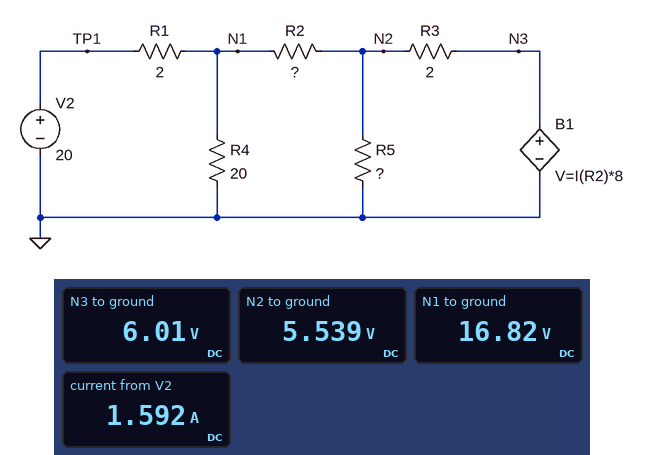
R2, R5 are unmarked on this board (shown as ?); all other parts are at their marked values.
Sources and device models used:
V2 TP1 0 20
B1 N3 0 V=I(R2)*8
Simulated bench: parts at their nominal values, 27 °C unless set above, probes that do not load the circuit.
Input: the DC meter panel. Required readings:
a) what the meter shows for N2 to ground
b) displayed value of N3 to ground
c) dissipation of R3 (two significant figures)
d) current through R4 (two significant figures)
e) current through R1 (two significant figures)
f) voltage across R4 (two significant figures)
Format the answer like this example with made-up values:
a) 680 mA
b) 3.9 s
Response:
a) 5.539 V
b) 6.01 V
c) 110 mW
d) 840 mA
e) 1.6 A
f) 17 V
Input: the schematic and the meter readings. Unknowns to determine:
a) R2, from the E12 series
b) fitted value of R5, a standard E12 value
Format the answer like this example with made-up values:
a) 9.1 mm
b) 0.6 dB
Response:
a) 15 Ω
b) 5.6 Ω
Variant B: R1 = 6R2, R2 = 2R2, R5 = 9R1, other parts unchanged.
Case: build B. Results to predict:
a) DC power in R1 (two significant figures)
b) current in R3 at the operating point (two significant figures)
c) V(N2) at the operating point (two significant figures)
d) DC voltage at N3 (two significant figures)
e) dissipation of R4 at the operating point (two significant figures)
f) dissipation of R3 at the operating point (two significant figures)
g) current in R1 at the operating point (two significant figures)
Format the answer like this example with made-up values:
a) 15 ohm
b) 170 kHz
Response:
a) 15 W
b) 100 mA
c) 8.3 V
d) 8.1 V
e) 5.5 W
f) 20 mW
g) 1.5 A
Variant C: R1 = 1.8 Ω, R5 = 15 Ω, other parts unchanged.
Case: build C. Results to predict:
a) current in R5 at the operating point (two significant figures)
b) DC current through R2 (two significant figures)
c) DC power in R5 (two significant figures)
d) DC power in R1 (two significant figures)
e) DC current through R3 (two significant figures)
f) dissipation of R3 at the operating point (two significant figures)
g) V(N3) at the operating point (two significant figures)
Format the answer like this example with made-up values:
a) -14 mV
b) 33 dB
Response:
a) 420 mA
b) 720 mA
c) 2.7 W
d) 4.5 W
e) 300 mA
f) 180 mW
g) 5.8 V
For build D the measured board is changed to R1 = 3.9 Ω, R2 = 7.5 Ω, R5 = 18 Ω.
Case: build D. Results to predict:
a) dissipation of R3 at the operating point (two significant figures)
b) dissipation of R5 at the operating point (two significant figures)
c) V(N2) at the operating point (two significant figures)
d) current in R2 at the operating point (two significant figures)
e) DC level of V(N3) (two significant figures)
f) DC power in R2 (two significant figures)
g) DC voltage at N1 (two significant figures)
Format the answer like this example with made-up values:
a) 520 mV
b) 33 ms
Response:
a) 360 mW
b) 3.2 W
c) 7.6 V
d) 850 mA
e) 6.8 V
f) 5.4 W
g) 14 V
